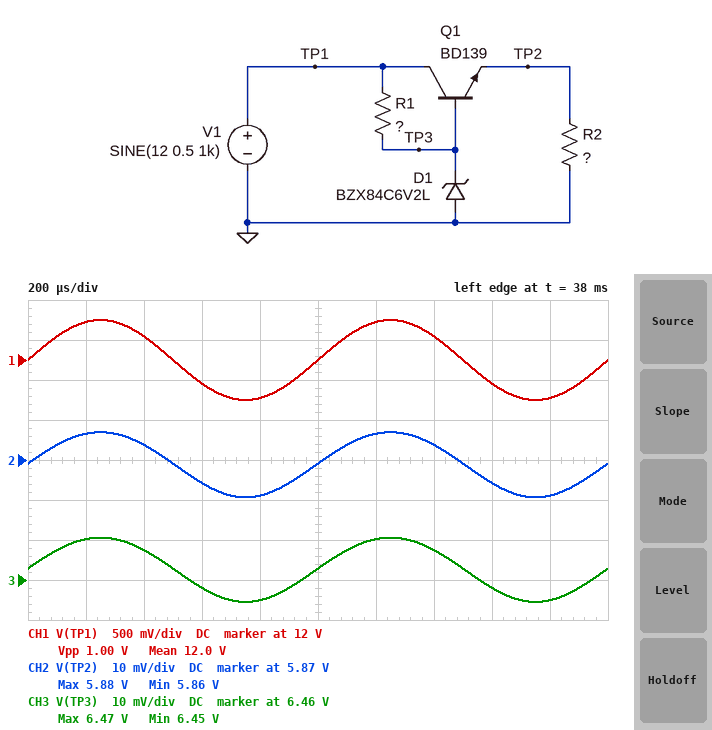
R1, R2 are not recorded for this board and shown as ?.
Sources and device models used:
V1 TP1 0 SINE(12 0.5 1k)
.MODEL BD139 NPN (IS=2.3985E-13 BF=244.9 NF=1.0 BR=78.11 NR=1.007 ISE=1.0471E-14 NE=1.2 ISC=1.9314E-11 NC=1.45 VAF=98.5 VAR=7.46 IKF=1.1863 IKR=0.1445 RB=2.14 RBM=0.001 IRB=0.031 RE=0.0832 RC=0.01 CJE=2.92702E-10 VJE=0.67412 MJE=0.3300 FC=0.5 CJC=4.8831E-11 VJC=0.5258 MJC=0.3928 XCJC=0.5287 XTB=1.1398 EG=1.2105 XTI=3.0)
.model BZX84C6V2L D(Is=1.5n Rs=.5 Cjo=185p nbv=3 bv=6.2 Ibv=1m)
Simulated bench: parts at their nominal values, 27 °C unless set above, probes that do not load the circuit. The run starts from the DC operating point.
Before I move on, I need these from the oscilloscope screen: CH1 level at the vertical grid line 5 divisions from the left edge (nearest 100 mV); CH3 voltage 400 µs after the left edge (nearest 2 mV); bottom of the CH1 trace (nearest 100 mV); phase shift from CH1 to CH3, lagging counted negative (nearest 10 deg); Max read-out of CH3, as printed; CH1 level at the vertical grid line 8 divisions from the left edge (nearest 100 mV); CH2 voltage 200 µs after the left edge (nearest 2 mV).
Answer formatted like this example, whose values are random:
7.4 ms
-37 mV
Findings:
12.0 V
6.468 V
11.5 V
0 deg
6.47 V
11.7 V
5.876 V
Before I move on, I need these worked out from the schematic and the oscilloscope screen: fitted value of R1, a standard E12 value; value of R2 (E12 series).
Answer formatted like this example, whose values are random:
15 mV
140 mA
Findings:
220 Ω
2.7 kΩ
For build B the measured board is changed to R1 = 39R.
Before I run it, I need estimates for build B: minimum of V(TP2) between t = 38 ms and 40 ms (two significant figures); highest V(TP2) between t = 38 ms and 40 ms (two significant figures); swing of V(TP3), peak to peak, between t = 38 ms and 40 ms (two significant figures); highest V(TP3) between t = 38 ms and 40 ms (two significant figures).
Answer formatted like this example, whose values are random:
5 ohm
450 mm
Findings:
6.0 V
6.1 V
27 mV
6.7 V
